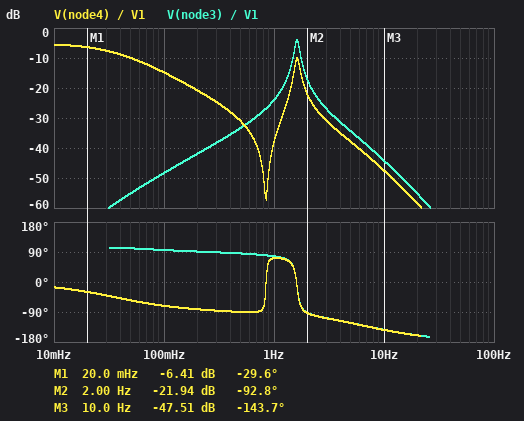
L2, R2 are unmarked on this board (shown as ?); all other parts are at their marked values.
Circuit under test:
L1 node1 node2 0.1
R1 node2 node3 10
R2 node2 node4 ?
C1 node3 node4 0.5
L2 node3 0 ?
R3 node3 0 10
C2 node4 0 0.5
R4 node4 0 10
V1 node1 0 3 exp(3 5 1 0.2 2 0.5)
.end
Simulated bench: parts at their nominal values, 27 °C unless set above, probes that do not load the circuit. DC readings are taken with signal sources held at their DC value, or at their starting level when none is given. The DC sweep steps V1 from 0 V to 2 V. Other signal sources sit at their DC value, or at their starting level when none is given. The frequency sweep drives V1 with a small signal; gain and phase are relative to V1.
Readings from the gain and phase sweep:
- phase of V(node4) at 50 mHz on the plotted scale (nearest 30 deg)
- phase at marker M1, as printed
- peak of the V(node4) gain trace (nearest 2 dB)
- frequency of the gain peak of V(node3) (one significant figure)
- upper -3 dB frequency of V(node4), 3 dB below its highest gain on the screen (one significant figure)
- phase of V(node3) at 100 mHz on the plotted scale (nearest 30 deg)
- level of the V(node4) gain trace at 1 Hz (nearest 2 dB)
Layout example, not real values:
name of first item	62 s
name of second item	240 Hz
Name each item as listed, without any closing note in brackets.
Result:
phase of V(node4) at 50 mHz on the plotted scale	-60 deg
phase at marker M1, as printed	-29.6 deg
peak of the V(node4) gain trace	-6 dB
frequency of the gain peak of V(node3)	2 Hz
upper -3 dB frequency of V(node4), 3 dB below its highest gain on the screen	40 mHz
phase of V(node3) at 100 mHz on the plotted scale	90 deg
level of the V(node4) gain trace at 1 Hz	-38 dB
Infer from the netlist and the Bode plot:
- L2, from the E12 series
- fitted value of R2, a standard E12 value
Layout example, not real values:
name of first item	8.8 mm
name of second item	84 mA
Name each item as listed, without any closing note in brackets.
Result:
L2, from the E12 series	39 mH
fitted value of R2, a standard E12 value	8.2 Ω
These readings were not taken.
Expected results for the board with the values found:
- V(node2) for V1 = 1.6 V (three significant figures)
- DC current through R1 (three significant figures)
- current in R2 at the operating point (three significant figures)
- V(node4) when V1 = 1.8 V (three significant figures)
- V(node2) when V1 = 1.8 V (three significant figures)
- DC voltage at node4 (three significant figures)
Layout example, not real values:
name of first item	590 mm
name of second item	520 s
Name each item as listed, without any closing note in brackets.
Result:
V(node2) for V1 = 1.6 V	1.60 V
DC current through R1	300 mA
current in R2 at the operating point	165 mA
V(node4) when V1 = 1.8 V	989 mV
V(node2) when V1 = 1.8 V	1.80 V
DC voltage at node4	1.65 V
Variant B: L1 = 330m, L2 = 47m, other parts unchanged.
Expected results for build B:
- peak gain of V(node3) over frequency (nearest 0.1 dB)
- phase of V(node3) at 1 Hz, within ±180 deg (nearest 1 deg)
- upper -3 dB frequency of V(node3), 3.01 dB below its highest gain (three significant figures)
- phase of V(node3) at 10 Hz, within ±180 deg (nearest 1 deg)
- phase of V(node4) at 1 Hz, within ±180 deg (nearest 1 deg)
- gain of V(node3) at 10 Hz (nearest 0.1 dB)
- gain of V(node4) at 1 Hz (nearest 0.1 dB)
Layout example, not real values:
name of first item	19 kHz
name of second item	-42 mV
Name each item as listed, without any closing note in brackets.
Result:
peak gain of V(node3) over frequency	-4.3 dB
phase of V(node3) at 1 Hz, within ±180 deg	59 deg
upper -3 dB frequency of V(node3), 3.01 dB below its highest gain	1.56 Hz
phase of V(node3) at 10 Hz, within ±180 deg	-167 deg
phase of V(node4) at 1 Hz, within ±180 deg	55 deg
gain of V(node3) at 10 Hz	-53.0 dB
gain of V(node4) at 1 Hz	-33.1 dB
